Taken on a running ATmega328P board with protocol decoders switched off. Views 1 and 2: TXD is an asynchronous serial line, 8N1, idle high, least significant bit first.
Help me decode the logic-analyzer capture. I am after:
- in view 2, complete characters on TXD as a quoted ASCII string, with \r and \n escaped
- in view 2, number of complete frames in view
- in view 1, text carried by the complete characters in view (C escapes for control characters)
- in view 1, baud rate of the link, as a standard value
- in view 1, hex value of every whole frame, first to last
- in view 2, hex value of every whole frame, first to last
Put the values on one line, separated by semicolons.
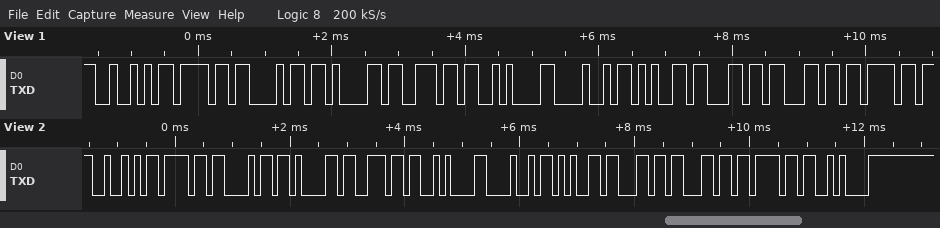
"Rohan\nHello\n"; 12; "Rohan\nHello"; 9600 baud; 0x52 0x6F 0x68 0x61 0x6E 0x0A 0x48 0x65 0x6C 0x6C 0x6F; 0x52 0x6F 0x68 0x61 0x6E 0x0A 0x48 0x65 0x6C 0x6C 0x6F 0x0A
